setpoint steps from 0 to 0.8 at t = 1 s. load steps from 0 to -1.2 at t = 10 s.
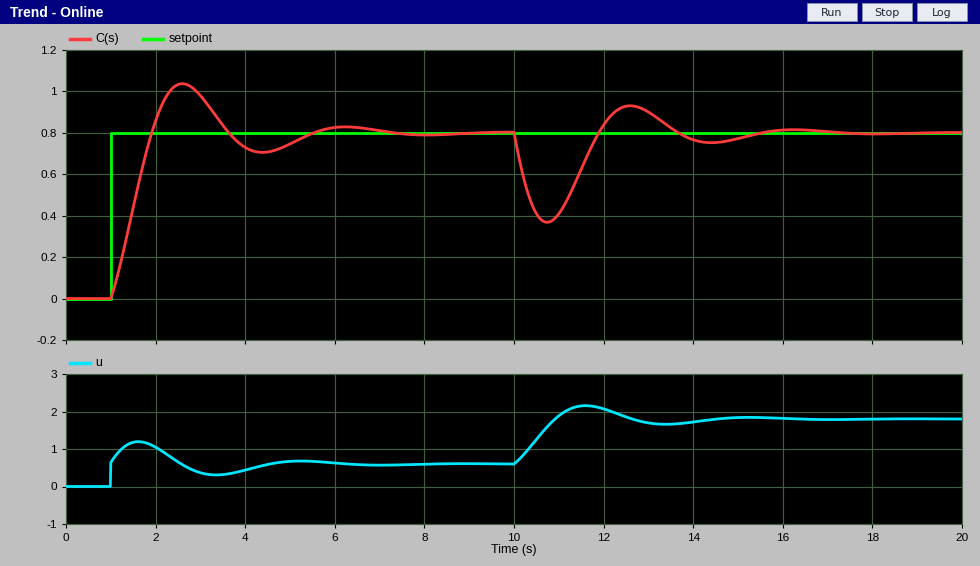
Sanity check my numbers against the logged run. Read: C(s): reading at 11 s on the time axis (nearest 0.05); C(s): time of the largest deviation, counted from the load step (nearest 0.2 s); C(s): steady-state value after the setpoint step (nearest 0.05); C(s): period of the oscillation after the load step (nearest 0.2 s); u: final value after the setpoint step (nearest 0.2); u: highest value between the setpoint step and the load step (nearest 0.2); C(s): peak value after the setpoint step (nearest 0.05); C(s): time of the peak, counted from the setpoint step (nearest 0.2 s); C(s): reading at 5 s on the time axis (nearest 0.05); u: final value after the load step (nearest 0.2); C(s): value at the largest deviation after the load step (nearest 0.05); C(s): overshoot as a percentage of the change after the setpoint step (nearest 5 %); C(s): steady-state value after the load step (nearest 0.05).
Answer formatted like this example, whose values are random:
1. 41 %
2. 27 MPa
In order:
1. 0.40
2. 0.8 s
3. 0.80
4. 3.6 s
5. 0.6
6. 1.2
7. 1.05
8. 1.6 s
9. 0.75
10. 1.8
11. 0.35
12. 30 %
13. 0.80
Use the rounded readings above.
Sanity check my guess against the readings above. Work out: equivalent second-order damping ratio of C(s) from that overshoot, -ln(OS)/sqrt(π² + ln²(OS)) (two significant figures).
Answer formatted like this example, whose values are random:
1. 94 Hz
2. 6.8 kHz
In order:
1. 0.36
